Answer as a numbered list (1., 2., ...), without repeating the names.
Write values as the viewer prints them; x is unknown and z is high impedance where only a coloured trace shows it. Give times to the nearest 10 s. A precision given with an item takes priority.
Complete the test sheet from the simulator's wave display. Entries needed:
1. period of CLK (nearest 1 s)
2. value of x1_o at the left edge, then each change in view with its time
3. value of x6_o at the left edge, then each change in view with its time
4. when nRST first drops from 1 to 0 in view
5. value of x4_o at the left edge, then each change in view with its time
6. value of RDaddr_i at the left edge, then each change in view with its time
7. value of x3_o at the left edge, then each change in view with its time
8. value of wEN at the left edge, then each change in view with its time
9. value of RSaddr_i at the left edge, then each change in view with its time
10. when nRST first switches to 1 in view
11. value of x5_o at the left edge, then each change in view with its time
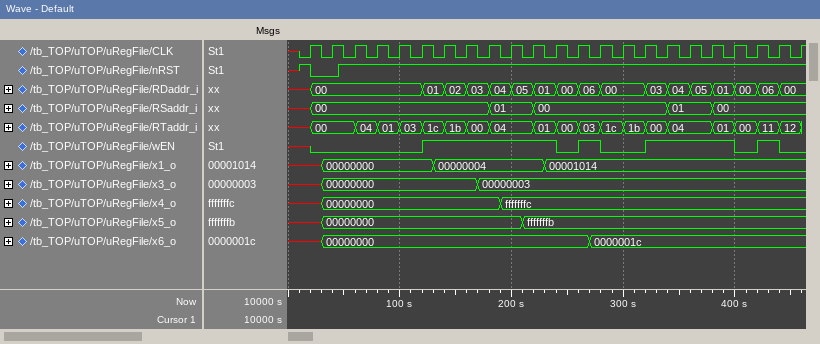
1. 20 s
2. x, 00000000 at 30 s, 00000004 at 130 s, 00001014 at 230 s
3. x, 00000000 at 30 s, 0000001c at 270 s
4. 20 s
5. x, 00000000 at 30 s, fffffffc at 190 s
6. x, 00 at 20 s, 01 at 120 s, 02 at 140 s, 03 at 160 s, 04 at 180 s, 05 at 200 s, 01 at 220 s, 00 at 240 s, 06 at 260 s, 00 at 280 s, 03 at 320 s, 04 at 340 s, 05 at 360 s, 01 at 380 s, 00 at 400 s, 06 at 420 s, 00 at 440 s
7. x, 00000000 at 30 s, 00000003 at 170 s
8. x, 0 at 20 s, 1 at 120 s, 0 at 240 s, 1 at 260 s, 0 at 280 s, 1 at 320 s, 0 at 400 s, 1 at 420 s, 0 at 440 s
9. x, 00 at 20 s, 01 at 180 s, 00 at 220 s, 01 at 340 s, 00 at 380 s
10. 10 s
11. x, 00000000 at 30 s, fffffffb at 210 s
